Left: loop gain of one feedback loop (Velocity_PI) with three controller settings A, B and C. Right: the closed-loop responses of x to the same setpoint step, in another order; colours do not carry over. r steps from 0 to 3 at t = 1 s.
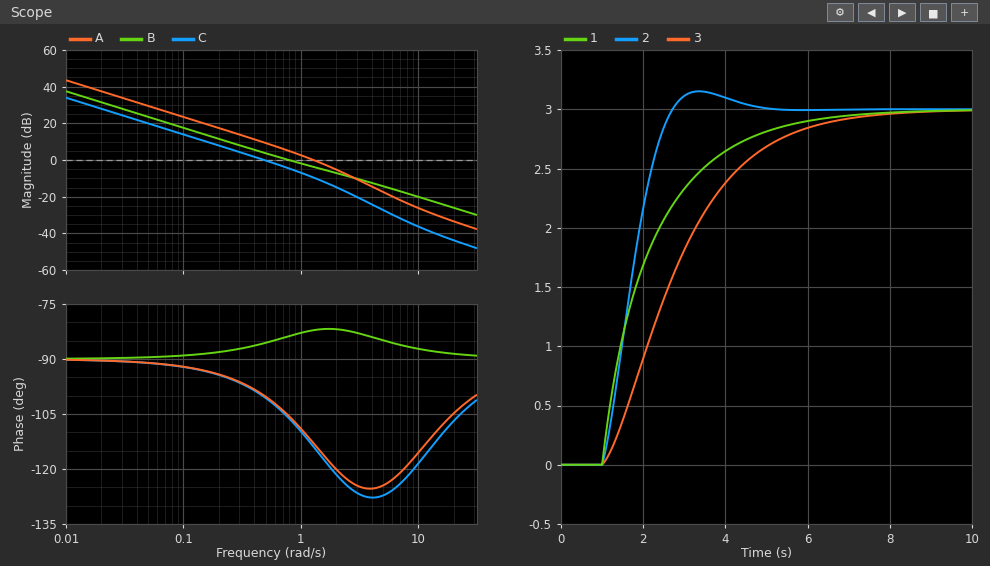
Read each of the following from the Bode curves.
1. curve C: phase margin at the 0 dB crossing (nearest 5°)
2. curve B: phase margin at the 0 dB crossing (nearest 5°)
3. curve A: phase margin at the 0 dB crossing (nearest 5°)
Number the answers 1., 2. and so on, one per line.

1. 80°
2. 95°
3. 65°
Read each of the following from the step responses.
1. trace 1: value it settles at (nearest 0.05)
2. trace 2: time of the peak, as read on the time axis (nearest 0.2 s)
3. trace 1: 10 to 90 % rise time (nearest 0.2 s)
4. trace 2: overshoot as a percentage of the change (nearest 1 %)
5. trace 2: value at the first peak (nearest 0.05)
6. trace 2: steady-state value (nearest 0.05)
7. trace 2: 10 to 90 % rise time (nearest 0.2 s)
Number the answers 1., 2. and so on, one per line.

1. 3.00
2. 3.4 s
3. 3.2 s
4. 5 %
5. 3.15
6. 3.00
7. 1.2 s
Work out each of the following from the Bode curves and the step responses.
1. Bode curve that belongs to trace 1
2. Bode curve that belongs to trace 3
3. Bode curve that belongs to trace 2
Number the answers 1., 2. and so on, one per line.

1. B
2. C
3. A
